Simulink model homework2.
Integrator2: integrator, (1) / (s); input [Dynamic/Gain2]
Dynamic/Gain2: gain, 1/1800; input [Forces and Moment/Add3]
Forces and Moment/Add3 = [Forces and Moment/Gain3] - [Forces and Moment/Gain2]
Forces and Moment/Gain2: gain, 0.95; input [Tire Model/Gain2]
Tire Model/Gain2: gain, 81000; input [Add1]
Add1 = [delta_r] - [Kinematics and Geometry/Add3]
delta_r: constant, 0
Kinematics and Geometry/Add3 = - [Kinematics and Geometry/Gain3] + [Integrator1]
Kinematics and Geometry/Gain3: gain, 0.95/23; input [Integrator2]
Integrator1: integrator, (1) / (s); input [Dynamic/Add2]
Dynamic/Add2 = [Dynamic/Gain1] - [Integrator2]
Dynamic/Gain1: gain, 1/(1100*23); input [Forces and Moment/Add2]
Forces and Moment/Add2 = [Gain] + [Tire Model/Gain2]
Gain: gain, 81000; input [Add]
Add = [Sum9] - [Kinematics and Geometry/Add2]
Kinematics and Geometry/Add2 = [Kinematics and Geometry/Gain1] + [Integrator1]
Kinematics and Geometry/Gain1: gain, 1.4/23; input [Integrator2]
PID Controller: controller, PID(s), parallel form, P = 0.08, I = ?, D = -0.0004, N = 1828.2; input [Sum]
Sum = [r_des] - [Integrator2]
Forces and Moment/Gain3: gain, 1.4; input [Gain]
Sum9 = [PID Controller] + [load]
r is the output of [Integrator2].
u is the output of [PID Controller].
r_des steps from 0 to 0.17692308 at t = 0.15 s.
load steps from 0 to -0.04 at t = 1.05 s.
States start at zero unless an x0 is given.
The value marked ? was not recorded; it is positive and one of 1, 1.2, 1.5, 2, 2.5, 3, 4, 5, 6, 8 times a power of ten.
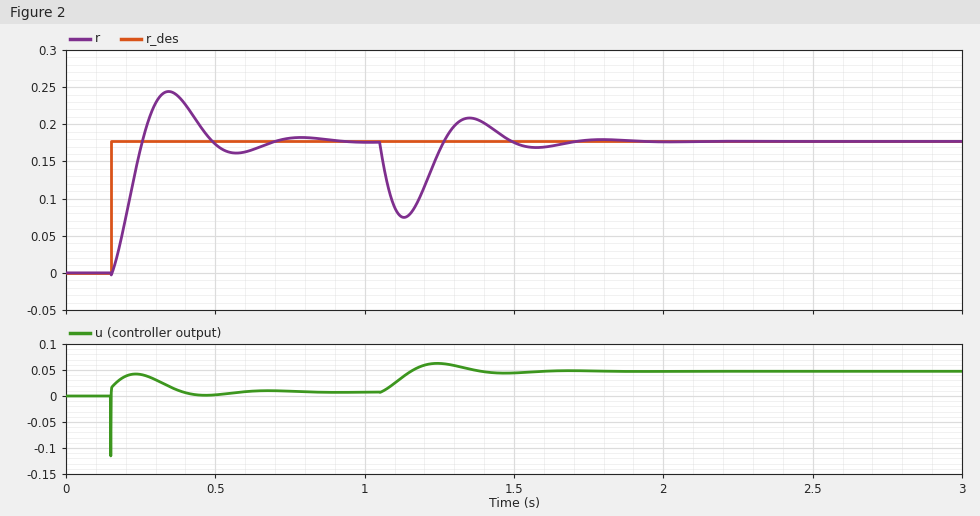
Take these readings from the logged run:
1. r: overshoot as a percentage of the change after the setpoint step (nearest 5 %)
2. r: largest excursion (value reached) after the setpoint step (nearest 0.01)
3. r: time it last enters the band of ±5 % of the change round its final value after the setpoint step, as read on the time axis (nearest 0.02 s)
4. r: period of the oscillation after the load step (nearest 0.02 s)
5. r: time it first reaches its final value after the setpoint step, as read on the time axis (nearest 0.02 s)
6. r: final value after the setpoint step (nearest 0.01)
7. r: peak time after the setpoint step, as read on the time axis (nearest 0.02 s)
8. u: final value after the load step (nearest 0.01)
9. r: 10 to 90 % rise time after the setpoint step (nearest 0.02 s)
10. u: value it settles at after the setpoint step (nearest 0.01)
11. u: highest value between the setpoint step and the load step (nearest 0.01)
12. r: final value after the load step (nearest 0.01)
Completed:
40 %
0.24
0.64 s
0.44 s
0.26 s
0.18
0.34 s
0.05
0.08 s
0.01
0.04
0.18
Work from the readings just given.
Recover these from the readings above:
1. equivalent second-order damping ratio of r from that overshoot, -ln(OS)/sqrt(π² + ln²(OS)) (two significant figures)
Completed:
0.28
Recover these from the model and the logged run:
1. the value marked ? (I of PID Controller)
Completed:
4
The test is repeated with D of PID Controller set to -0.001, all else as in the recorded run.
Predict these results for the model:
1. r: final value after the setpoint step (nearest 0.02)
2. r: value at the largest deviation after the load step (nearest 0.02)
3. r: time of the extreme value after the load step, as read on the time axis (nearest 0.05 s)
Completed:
0.18
0.08
1.15 s
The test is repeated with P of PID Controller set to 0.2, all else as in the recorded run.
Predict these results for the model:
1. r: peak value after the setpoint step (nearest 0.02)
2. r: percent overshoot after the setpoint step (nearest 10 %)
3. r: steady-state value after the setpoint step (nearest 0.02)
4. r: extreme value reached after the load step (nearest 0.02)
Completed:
0.22
20 %
0.18
0.10
